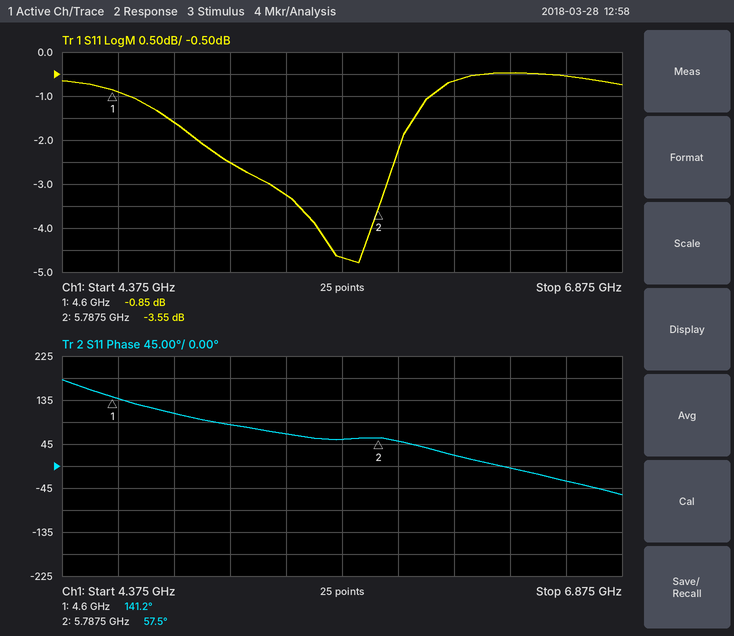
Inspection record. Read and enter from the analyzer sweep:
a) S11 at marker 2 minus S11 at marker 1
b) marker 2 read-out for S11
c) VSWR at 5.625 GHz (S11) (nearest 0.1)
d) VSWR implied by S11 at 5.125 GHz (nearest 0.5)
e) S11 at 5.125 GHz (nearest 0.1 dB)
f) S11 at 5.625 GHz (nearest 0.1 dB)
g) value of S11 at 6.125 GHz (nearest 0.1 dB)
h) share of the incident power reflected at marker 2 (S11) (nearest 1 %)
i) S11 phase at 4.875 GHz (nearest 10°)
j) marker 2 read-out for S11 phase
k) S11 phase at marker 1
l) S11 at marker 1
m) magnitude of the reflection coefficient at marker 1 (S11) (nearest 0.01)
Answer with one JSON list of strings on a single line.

["-2.70 dB", "-3.55 dB", "3.8", "7.0", "-2.5 dB", "-4.7 dB", "-0.7 dB", "44 %", "110°", "57.5°", "141.2°", "-0.85 dB", "0.91"]
